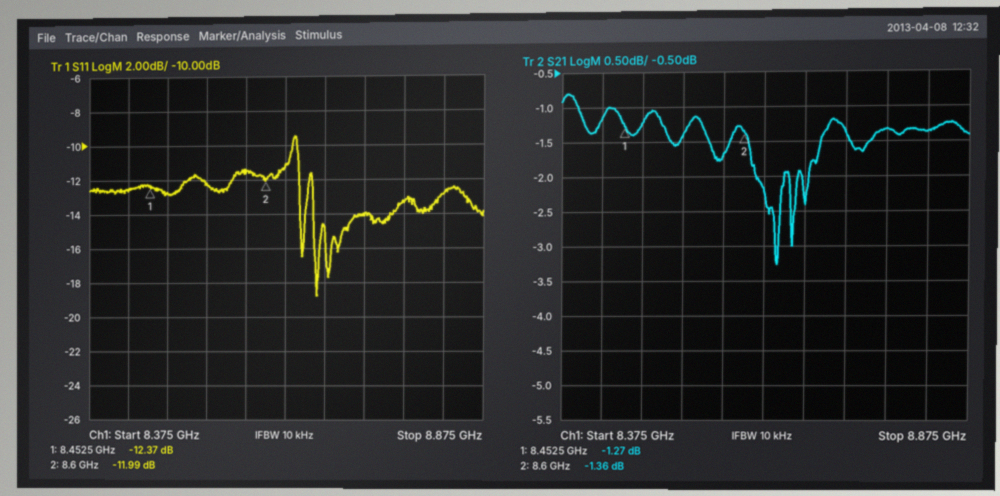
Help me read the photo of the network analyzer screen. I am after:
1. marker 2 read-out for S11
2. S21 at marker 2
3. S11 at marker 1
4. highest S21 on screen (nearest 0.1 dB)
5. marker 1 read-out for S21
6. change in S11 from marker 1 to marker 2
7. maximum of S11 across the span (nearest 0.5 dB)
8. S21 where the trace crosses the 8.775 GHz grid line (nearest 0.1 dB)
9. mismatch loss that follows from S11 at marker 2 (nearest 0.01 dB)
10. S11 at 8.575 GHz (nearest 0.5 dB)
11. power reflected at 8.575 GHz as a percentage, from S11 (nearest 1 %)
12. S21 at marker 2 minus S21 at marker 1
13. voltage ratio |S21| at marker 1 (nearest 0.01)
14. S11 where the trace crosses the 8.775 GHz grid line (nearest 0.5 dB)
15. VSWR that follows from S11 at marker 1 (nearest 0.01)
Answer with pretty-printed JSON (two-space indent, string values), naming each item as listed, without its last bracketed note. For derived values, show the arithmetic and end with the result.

{
  "marker 2 read-out for S11": "-11.99 dB",
  "S21 at marker 2": "-1.36 dB",
  "S11 at marker 1": "-12.37 dB",
  "highest S21 on screen": "-0.8 dB",
  "marker 1 read-out for S21": "-1.27 dB",
  "change in S11 from marker 1 to marker 2": "-11.99 − (-12.37) = 0.38 dB",
  "maximum of S11 across the span": "-9.5 dB",
  "S21 where the trace crosses the 8.775 GHz grid line": "-1.3 dB",
  "mismatch loss that follows from S11 at marker 2": "−10 log10(1 − 10^(-11.99/10)) ≈ 0.28 dB",
  "S11 at 8.575 GHz": "-11.5 dB",
  "power reflected at 8.575 GHz as a percentage, from S11": "10^(-11.5/10) ≈ 7 %",
  "S21 at marker 2 minus S21 at marker 1": "-1.36 − (-1.27) = -0.09 dB",
  "voltage ratio |S21| at marker 1": "10^(-1.27/20) ≈ 0.86",
  "S11 where the trace crosses the 8.775 GHz grid line": "-13.5 dB",
  "VSWR that follows from S11 at marker 1": "(1 + 0.2407)/(1 − 0.2407) ≈ 1.63"
}
